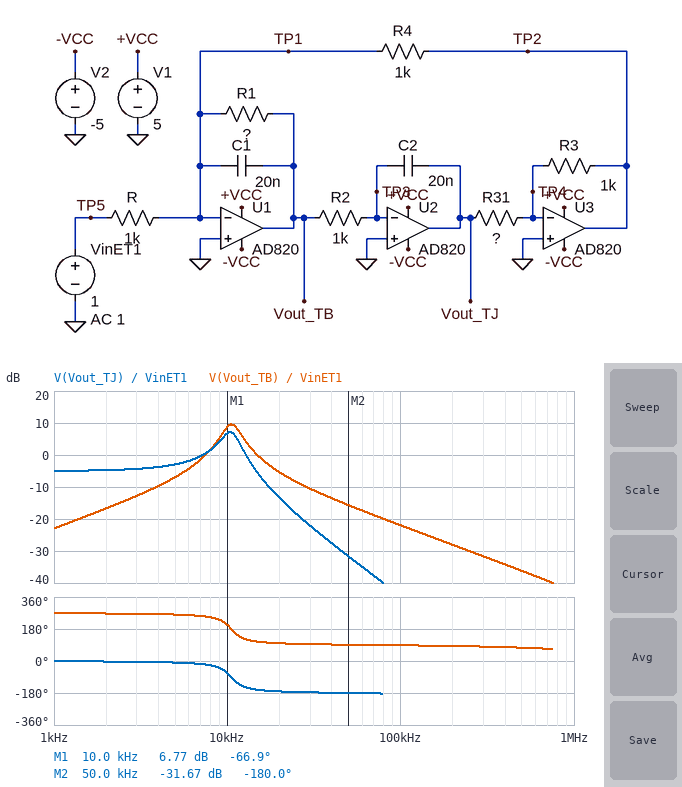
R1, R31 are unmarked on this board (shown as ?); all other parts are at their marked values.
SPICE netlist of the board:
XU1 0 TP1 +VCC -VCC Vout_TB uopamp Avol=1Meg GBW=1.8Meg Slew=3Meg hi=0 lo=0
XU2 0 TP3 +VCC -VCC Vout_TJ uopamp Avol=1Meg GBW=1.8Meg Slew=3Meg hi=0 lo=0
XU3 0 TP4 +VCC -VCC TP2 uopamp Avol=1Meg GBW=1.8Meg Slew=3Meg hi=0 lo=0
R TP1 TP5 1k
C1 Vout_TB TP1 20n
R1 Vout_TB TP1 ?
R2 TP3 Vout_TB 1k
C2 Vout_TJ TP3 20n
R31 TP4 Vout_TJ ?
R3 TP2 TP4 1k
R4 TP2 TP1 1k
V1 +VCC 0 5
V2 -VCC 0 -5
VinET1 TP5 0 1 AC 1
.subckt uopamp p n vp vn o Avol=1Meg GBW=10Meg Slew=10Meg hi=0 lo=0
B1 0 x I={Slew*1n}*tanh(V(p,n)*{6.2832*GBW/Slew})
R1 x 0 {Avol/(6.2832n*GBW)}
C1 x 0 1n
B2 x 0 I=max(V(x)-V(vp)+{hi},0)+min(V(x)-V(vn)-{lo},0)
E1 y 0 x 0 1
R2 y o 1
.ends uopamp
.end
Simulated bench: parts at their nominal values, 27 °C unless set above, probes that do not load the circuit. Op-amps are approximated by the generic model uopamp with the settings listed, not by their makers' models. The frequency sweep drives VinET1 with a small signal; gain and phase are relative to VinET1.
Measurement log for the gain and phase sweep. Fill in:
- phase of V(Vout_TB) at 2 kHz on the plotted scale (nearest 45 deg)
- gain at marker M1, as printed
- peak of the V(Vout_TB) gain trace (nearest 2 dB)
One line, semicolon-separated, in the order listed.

270 deg; 6.77 dB; 10 dB
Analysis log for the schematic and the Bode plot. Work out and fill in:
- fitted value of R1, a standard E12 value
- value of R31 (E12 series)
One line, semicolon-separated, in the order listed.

2.7 kΩ; 560 Ω
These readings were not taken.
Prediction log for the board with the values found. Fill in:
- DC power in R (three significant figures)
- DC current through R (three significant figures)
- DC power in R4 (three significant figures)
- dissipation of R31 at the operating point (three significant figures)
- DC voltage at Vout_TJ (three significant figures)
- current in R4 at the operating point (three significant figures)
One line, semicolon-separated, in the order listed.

1.00 mW; 1.00 mA; 1.00 mW; 560 µW; 560 mV; 1.00 mA
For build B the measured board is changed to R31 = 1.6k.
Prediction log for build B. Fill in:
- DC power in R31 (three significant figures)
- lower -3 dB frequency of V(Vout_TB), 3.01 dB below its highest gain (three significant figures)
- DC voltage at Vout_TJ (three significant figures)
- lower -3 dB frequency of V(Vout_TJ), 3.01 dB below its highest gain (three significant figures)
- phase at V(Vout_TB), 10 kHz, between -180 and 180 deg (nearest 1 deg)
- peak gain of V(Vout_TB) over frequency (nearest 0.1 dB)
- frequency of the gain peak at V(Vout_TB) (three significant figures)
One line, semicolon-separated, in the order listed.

1.60 mW; 4.99 kHz; 1.60 V; 4.21 kHz; 115 deg; 8.9 dB; 6.25 kHz
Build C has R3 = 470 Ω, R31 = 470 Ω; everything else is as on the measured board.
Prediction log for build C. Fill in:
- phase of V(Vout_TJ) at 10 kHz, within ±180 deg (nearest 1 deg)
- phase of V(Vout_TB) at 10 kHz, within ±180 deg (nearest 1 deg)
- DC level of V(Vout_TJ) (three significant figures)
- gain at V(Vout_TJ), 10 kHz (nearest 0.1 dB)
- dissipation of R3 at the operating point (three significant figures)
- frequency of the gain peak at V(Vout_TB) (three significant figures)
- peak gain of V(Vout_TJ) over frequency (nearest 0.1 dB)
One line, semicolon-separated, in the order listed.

-144 deg; 126 deg; 1.00 V; 2.5 dB; 2.13 mW; 7.90 kHz; 9.2 dB
